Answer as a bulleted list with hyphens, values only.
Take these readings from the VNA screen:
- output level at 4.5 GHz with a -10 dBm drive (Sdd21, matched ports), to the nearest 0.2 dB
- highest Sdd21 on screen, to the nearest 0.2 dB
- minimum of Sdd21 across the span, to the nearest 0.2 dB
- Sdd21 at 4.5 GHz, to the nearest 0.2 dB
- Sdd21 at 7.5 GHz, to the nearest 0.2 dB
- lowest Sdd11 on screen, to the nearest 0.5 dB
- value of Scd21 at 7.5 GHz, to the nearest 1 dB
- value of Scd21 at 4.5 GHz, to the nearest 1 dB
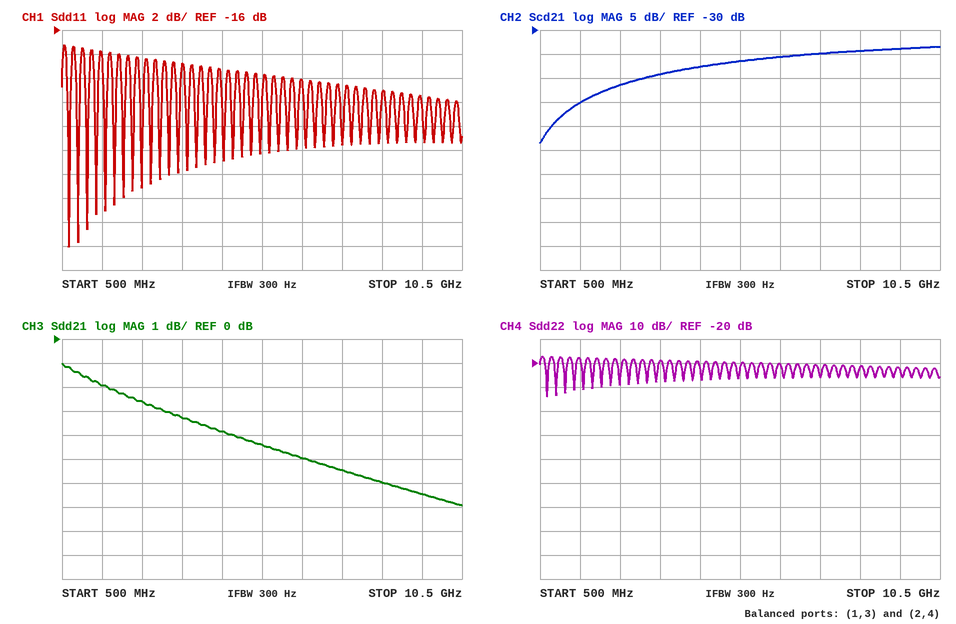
- -13.8 dBm
- -1.0 dB
- -7.0 dB
- -3.8 dB
- -5.4 dB
- -34.0 dB
- -35 dB
- -38 dB
